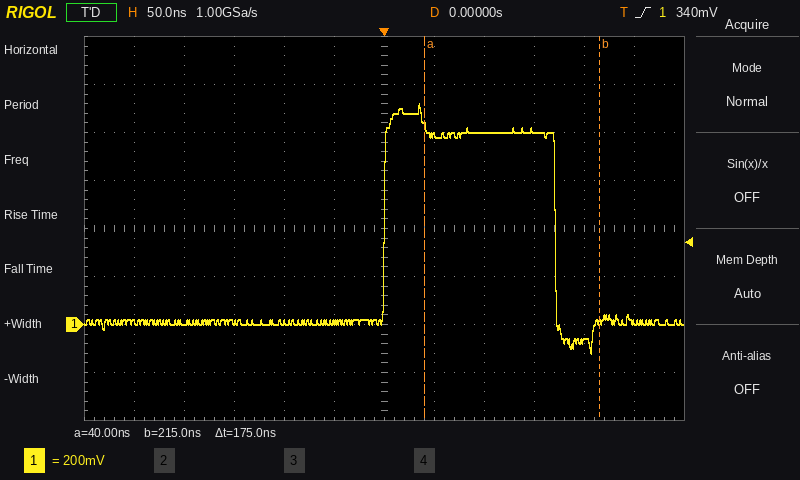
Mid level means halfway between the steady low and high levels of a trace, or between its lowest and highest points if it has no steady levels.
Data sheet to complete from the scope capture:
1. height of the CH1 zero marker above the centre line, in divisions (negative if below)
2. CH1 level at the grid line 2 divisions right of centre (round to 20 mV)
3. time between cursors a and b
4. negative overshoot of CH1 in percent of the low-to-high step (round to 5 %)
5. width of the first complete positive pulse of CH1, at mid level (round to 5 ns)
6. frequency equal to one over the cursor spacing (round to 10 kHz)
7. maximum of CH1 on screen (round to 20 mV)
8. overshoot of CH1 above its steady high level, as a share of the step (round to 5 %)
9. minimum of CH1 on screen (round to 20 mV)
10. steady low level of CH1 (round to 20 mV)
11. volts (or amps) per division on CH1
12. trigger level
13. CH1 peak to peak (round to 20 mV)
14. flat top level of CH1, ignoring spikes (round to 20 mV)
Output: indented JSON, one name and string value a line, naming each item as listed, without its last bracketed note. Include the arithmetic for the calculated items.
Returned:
{
  "height of the CH1 zero marker above the centre line, in divisions": "-2.0 div",
  "CH1 level at the grid line 2 divisions right of centre": "800 mV",
  "time between cursors a and b": "175 ns",
  "negative overshoot of CH1 in percent of the low-to-high step": "15 %",
  "width of the first complete positive pulse of CH1, at mid level": "170 ns",
  "frequency equal to one over the cursor spacing": "1 / 175 ns ≈ 5.71 MHz",
  "maximum of CH1 on screen": "920 mV",
  "overshoot of CH1 above its steady high level, as a share of the step": "15 %",
  "minimum of CH1 on screen": "-120 mV",
  "steady low level of CH1": "0 mV",
  "volts (or amps) per division on CH1": "200 mV",
  "trigger level": "340 mV",
  "CH1 peak to peak": "920 mV − (-120 mV) = 1.04 V",
  "flat top level of CH1, ignoring spikes": "800 mV"
}
